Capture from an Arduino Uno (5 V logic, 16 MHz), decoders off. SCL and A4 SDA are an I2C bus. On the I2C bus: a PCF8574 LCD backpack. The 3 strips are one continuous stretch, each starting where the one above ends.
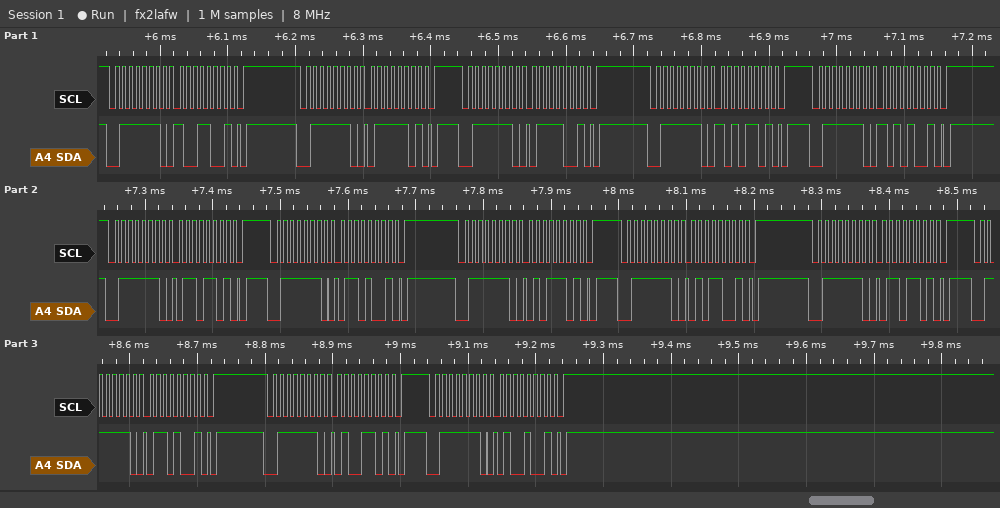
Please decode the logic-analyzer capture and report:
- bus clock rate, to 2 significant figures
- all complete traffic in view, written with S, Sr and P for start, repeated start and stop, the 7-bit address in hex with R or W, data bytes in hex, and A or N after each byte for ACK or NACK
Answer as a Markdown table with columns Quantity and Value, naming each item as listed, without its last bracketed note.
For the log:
| Quantity | Value |
|---|---|
| bus clock rate, to 2 significant figures | 100 kHz |
| all complete traffic in view, written with S, Sr and P for start, repeated start and stop, the 7-bit address in hex with R or W, data bytes in hex, and A or N after each byte for ACK or NACK | S 3FW A 99 A P S 3FW A 7D A P S 3FW A 79 A P S 3FW A AD A P S 3FW A A9 A P S 3FW A 6D A P S 3FW A 69 A P S 3FW A 5D A P S 3FW A 59 A P S 3FW A 6D A P S 3FW A 69 A P S 3FW A 4D A P S 3FW A 49 A P |
